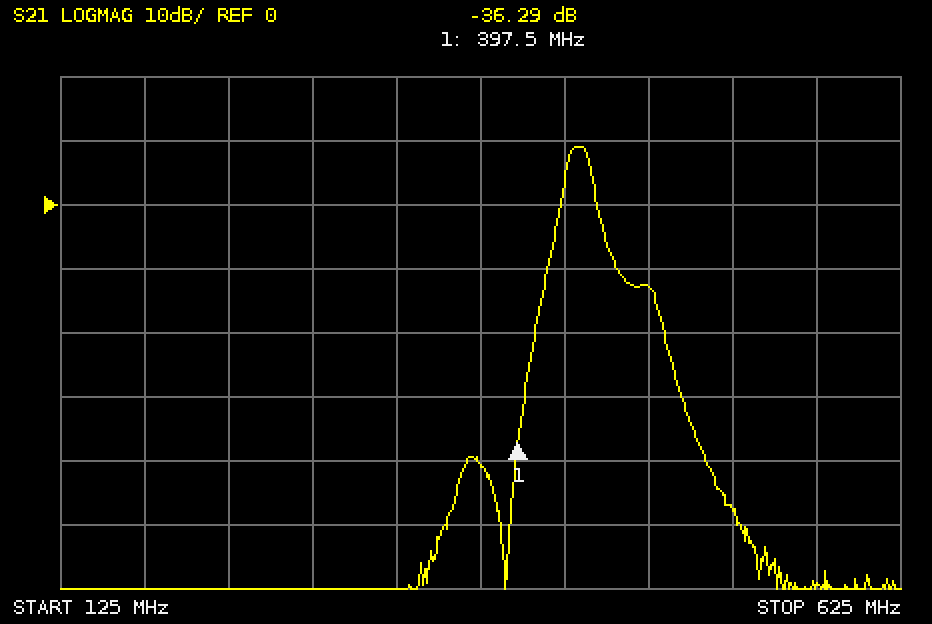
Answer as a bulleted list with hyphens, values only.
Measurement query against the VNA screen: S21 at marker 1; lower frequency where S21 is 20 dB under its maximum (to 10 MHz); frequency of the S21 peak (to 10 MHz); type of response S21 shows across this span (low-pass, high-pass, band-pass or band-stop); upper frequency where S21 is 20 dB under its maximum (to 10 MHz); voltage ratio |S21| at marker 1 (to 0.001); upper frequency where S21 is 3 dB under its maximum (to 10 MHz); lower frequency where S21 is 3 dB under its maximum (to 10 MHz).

- -36.29 dB
- 410 MHz
- 430 MHz
- band-pass
- 460 MHz
- 0.015
- 440 MHz
- 430 MHz
